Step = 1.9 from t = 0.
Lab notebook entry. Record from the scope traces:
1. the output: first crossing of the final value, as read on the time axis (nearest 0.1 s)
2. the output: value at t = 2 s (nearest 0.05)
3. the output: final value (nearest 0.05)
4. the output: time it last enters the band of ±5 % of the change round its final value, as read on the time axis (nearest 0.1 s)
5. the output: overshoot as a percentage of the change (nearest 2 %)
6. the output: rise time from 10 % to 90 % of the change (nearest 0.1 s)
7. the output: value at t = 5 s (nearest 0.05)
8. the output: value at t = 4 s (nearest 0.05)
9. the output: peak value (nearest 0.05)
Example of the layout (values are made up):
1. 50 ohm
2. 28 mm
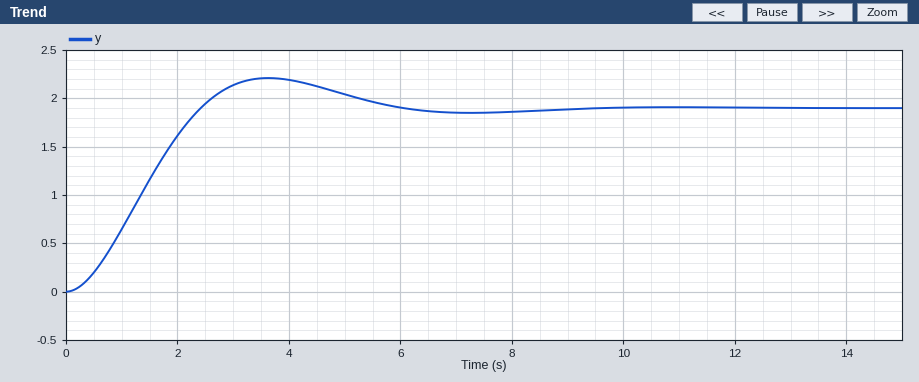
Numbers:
1. 2.4 s
2. 1.60
3. 1.90
4. 5.3 s
5. 16 %
6. 1.6 s
7. 2.05
8. 2.20
9. 2.20
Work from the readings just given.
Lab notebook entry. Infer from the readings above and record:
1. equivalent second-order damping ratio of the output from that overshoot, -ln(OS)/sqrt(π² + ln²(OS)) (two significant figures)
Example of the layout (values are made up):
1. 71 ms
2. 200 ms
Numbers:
1. 0.50
